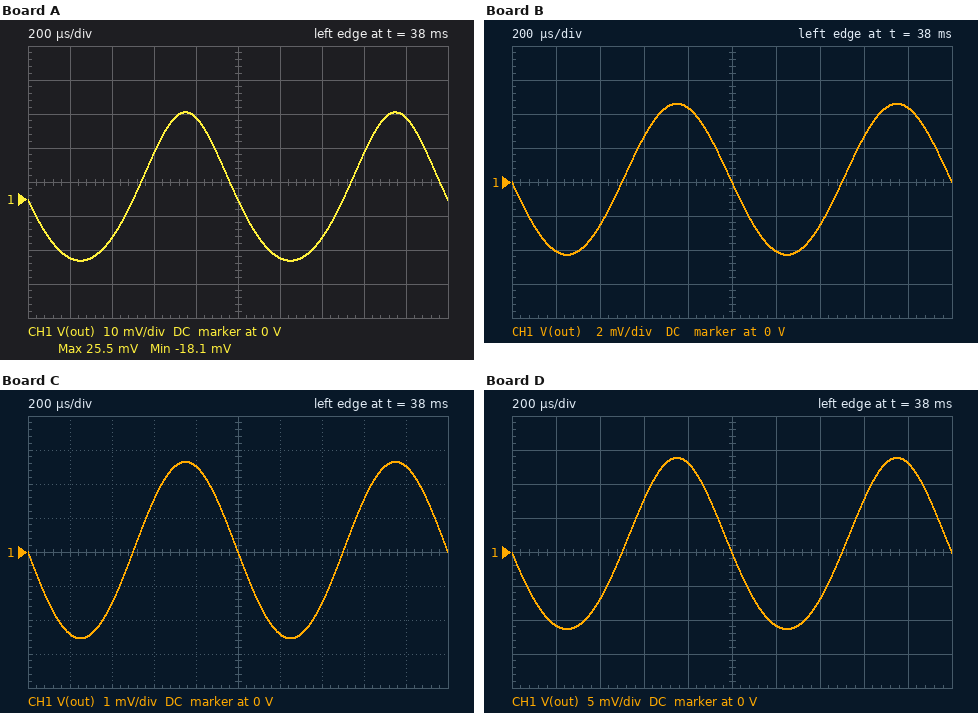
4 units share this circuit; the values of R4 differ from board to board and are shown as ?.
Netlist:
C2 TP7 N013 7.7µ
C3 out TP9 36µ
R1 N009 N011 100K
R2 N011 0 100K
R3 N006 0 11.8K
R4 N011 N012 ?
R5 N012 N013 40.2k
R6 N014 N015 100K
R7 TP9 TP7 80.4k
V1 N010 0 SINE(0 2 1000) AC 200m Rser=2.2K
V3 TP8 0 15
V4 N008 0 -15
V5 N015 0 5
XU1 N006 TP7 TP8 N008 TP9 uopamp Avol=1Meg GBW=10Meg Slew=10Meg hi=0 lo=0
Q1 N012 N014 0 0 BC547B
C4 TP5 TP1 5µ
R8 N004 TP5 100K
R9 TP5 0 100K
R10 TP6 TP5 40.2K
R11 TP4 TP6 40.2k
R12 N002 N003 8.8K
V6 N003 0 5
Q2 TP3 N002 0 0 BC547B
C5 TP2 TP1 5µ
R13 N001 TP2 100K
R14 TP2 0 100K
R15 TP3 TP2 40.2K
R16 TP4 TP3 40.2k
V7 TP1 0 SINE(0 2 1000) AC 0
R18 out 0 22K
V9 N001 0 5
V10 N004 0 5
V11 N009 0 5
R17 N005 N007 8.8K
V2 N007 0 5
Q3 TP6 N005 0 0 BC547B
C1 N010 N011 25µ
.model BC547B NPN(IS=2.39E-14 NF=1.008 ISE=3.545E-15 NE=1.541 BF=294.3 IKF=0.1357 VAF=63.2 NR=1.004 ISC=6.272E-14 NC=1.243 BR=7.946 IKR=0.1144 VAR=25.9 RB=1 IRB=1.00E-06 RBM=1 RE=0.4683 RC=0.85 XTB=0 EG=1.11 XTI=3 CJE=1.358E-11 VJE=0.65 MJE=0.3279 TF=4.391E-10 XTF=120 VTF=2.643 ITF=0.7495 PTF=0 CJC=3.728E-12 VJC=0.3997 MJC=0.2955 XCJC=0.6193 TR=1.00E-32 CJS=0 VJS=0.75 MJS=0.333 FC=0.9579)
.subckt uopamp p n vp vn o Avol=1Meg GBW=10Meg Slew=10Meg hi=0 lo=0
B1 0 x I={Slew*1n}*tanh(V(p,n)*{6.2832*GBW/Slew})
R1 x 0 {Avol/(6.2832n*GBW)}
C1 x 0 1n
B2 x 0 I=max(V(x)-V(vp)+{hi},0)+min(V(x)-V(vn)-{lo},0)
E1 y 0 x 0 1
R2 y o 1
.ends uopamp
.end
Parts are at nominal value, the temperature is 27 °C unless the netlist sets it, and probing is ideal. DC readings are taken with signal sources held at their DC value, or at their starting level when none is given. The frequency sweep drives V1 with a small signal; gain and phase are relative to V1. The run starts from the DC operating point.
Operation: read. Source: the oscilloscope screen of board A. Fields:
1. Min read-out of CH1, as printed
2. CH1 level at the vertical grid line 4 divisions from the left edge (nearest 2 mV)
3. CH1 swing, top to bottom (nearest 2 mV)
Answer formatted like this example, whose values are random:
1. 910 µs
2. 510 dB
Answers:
1. -18.1 mV
2. 24 mV
3. 44 mV
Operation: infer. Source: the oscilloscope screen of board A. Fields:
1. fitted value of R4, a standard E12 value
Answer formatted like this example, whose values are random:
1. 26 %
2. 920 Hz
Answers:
1. 12 kΩ
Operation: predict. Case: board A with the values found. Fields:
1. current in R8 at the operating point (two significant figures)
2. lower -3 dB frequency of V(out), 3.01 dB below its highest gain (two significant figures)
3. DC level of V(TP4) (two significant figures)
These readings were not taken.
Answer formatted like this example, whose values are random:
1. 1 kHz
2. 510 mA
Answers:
1. 39 µA
2. 850 mHz
3. 7.0 mV
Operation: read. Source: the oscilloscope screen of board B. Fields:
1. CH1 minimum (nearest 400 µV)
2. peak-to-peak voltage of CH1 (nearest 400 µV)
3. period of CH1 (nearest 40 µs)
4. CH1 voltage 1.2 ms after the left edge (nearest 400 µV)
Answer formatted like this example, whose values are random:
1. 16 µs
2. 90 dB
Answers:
1. -4.4 mV
2. 8.8 mV
3. 1.00 ms
4. -4.0 mV
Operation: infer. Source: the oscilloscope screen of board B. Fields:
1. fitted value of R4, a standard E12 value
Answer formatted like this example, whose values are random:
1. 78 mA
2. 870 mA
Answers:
1. 68 kΩ
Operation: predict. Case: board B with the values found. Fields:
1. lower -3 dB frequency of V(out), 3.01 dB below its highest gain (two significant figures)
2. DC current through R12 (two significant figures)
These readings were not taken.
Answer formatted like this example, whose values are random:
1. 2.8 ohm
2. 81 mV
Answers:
1. 640 mHz
2. 490 µA
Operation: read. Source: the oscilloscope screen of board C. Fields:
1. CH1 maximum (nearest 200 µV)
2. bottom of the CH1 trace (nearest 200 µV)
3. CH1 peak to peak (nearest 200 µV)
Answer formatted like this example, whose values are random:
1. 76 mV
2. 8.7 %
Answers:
1. 2.6 mV
2. -2.6 mV
3. 5.2 mV
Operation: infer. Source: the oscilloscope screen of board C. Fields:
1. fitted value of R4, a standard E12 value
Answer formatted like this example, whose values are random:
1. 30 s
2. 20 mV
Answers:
1. 120 kΩ
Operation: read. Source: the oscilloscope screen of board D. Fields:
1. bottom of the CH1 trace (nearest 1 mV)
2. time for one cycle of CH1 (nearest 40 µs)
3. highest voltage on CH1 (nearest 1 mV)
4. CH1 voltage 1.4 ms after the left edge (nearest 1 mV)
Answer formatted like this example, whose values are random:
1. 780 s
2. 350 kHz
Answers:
1. -11 mV
2. 1.00 ms
3. 14 mV
4. -7 mV
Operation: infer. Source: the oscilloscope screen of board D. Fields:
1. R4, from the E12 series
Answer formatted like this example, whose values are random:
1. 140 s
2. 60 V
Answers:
1. 22 kΩ
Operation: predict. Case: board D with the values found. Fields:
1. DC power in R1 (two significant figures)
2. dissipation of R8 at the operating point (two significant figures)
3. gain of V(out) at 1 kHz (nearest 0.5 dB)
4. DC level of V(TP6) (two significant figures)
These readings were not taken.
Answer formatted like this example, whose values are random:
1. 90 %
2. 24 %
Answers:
1. 180 µW
2. 150 µW
3. -44.0 dB
4. 7.0 mV
